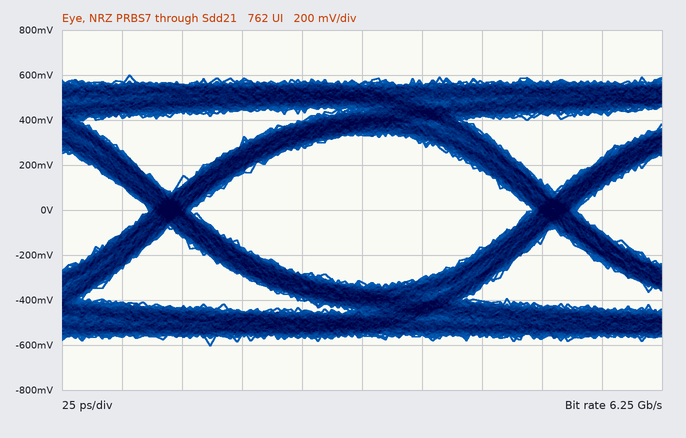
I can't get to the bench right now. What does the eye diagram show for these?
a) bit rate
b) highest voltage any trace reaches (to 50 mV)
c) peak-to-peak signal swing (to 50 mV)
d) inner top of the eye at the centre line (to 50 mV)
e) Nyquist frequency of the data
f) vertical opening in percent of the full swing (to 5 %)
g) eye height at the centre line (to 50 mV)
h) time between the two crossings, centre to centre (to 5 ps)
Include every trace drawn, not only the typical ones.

6.25 Gb/s
600 mV
1.20 V
350 mV
3.125 GHz
55 %
650 mV
160 ps
